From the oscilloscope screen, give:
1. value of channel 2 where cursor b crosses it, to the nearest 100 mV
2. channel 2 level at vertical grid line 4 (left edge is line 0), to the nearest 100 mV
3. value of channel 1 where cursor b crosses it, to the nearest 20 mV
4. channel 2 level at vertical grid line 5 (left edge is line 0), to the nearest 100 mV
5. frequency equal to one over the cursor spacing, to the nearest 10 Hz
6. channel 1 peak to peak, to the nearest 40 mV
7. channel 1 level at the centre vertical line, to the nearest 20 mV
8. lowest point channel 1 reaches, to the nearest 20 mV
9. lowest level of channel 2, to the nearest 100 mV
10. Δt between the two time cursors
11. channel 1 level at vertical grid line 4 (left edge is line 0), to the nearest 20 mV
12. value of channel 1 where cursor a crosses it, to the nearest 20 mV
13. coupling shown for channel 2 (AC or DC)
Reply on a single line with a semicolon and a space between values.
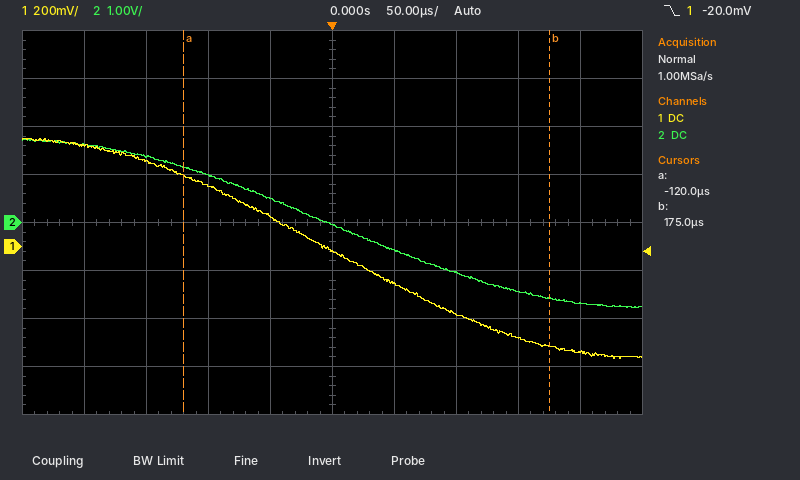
-1.6 V; 500 mV; -420 mV; 0.0 V; 3.39 kHz; 920 mV; -20 mV; -460 mV; -1.8 V; 295 µs; 120 mV; 300 mV; DC
